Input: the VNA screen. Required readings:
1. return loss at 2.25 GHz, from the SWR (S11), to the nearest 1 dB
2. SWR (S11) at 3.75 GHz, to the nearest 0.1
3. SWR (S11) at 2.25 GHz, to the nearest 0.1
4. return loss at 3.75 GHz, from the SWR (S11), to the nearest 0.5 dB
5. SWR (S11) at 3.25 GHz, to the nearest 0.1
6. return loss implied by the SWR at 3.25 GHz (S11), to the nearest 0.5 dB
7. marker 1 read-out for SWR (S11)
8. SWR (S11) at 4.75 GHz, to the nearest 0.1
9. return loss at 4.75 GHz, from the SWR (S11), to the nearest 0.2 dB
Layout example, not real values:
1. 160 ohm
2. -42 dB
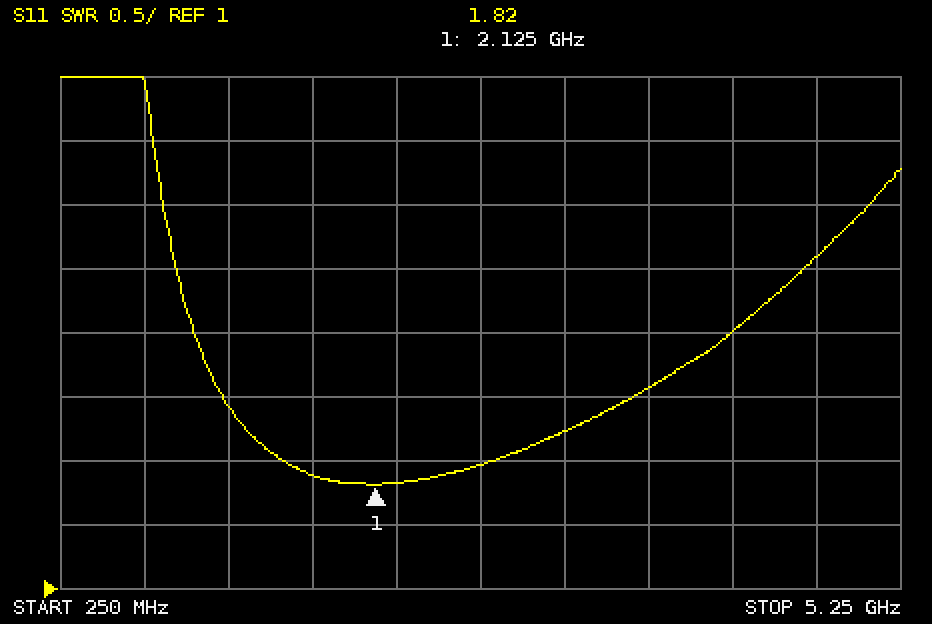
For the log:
1. 11 dB
2. 2.6
3. 1.8
4. 7.0 dB
5. 2.2
6. 8.5 dB
7. 1.82
8. 3.6
9. 5.0 dB
